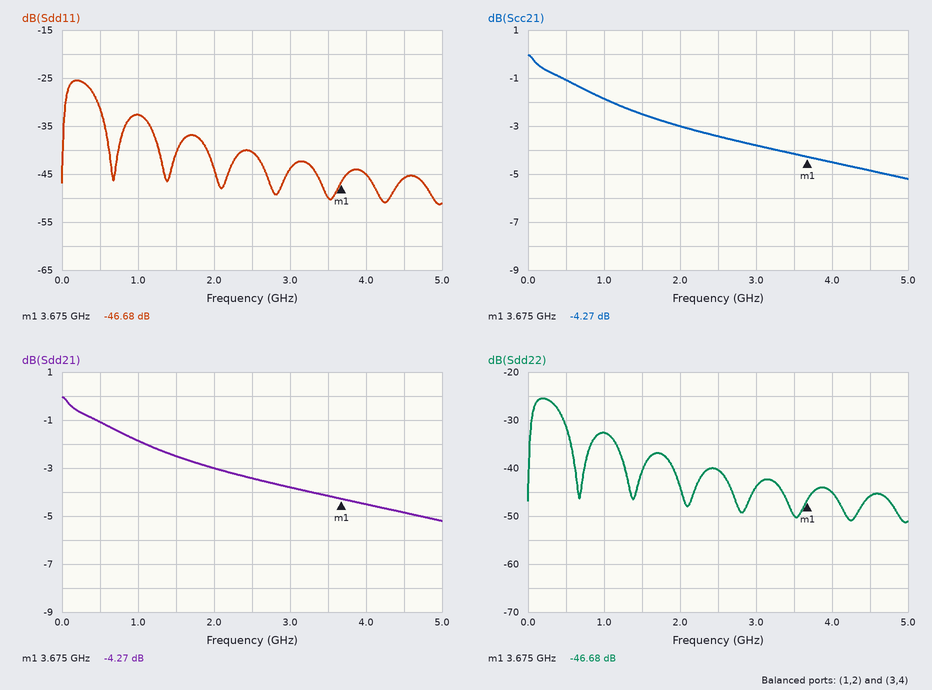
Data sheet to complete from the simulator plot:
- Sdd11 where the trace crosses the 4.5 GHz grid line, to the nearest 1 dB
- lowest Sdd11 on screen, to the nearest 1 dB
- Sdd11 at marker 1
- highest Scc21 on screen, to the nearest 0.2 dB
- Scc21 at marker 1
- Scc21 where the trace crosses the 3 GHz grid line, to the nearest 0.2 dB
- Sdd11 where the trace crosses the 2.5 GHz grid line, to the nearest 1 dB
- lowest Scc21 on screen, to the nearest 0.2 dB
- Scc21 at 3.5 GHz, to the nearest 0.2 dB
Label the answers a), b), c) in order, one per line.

a) -46 dB
b) -51 dB
c) -46.68 dB
d) 0.0 dB
e) -4.27 dB
f) -3.8 dB
g) -40 dB
h) -5.2 dB
i) -4.2 dB
